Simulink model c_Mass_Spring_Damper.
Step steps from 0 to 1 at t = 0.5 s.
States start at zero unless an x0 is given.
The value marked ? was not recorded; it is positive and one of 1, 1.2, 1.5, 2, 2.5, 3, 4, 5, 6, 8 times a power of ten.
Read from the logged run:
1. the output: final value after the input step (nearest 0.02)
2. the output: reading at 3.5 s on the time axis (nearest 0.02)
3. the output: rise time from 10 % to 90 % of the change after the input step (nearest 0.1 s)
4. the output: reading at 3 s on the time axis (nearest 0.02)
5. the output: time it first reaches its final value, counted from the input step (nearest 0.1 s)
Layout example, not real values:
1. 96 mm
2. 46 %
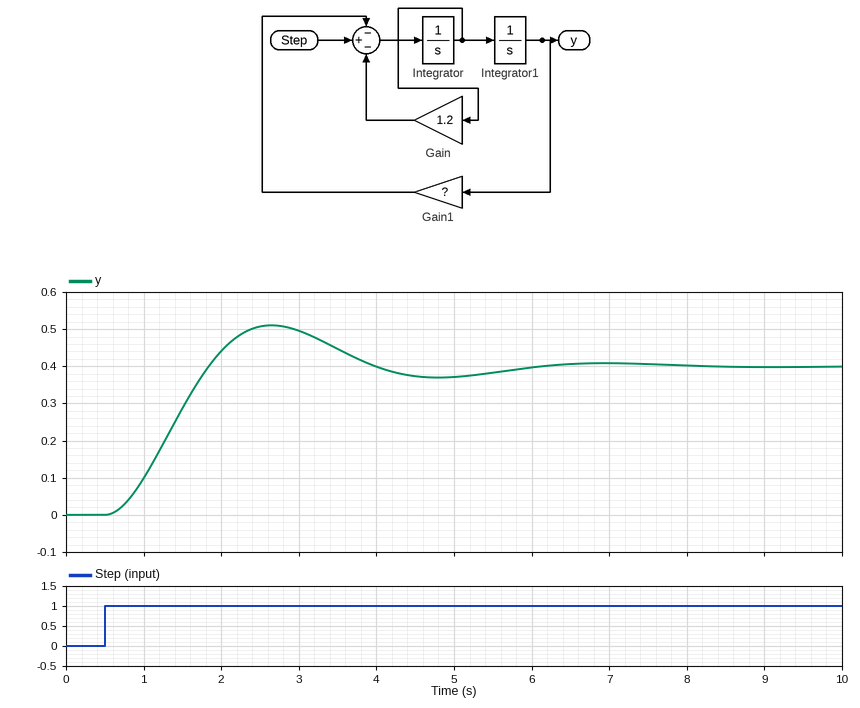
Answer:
1. 0.40
2. 0.44
3. 0.9 s
4. 0.50
5. 1.3 s
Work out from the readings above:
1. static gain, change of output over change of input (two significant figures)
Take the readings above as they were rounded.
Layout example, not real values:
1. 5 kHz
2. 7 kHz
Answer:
1. 0.40
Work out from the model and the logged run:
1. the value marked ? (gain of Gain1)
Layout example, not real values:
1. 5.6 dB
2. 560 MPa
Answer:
1. 2.5
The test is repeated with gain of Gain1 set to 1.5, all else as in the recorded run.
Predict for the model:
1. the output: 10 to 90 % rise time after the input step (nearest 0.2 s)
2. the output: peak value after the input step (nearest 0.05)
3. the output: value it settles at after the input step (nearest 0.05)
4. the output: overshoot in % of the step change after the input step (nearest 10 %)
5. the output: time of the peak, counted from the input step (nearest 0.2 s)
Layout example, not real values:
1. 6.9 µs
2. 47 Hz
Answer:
1. 1.4 s
2. 0.80
3. 0.65
4. 20 %
5. 3.0 s
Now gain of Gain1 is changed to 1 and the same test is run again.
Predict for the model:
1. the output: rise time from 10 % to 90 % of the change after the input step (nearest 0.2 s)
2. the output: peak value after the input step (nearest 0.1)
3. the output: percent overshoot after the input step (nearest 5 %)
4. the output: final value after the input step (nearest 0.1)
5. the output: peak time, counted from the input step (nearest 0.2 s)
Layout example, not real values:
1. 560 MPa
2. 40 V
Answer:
1. 1.8 s
2. 1.1
3. 10 %
4. 1.0
5. 4.0 s
